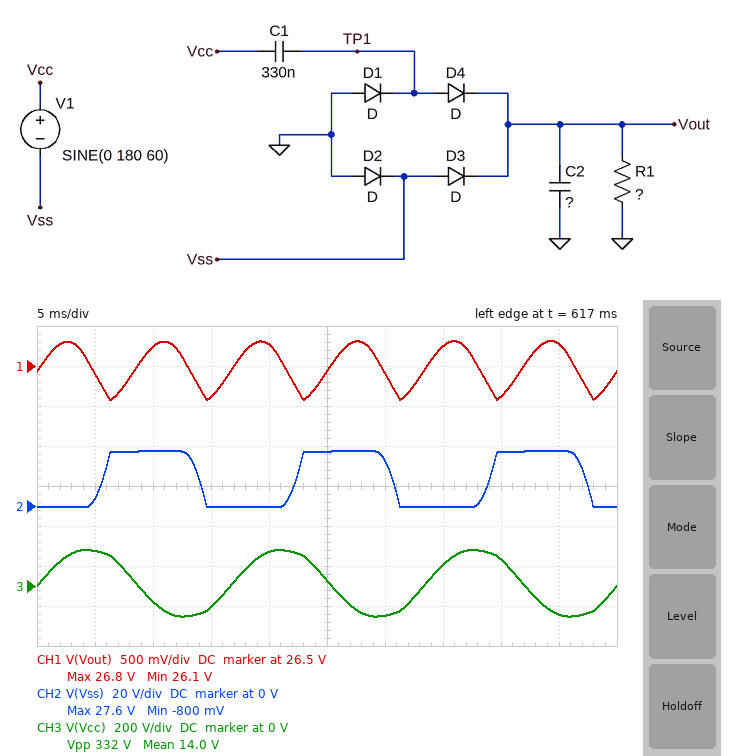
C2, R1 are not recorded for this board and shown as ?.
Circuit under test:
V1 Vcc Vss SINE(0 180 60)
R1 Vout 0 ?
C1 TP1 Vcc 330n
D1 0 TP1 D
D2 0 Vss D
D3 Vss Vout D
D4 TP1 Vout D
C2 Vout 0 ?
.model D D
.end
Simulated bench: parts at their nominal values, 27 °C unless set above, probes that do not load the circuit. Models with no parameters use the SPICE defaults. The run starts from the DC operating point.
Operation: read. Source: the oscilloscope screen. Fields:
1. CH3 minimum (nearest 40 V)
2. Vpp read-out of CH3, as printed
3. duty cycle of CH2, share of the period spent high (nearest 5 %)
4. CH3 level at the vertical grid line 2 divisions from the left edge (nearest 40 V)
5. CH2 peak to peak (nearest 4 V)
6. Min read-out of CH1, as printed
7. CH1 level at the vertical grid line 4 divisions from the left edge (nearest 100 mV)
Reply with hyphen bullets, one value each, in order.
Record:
- -160 V
- 332 V
- 50 %
- -80 V
- 28 V
- 26.1 V
- 26.8 V
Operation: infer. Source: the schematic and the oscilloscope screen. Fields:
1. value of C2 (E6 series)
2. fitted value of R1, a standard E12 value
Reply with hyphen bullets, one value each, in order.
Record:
- 47 µF
- 2.2 kΩ
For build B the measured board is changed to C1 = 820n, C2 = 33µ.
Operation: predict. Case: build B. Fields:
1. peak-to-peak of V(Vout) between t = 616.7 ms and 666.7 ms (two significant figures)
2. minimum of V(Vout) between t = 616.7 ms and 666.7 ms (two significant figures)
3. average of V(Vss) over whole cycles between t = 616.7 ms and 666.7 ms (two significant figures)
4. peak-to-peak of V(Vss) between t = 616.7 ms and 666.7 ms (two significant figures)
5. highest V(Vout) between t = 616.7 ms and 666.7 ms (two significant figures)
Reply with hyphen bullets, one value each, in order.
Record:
- 2.7 V
- 52 V
- 27 V
- 56 V
- 55 V
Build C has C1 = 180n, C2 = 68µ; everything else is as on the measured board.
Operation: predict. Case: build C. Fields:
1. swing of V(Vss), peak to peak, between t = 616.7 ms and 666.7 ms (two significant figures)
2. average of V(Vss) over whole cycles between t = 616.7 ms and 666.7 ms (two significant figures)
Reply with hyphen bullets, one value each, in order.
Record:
- 17 V
- 7.7 V
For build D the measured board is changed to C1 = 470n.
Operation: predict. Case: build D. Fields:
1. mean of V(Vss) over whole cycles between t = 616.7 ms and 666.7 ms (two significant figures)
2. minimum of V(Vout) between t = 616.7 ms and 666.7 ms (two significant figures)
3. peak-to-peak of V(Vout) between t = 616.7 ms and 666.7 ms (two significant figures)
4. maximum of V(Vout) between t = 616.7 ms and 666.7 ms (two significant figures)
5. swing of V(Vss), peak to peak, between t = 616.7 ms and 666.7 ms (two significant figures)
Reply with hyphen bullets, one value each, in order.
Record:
- 18 V
- 35 V
- 1.1 V
- 36 V
- 37 V
